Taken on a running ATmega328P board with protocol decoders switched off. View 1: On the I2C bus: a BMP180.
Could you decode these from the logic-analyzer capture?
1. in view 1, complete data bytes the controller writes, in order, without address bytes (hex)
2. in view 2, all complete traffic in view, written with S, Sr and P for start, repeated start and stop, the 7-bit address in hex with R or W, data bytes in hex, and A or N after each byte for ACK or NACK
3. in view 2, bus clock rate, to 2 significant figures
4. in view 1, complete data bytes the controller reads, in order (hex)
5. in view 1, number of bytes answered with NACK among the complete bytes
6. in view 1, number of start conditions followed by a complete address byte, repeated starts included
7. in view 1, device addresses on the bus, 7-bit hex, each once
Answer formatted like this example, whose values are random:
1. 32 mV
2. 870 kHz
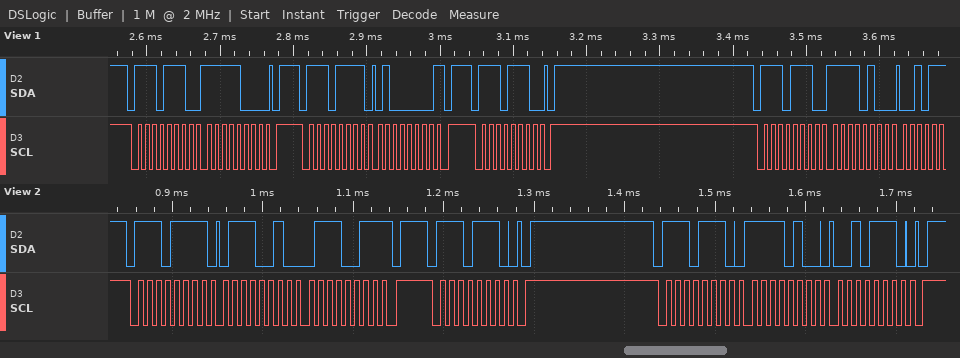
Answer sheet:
1. F8 F4
2. S 77R A 72 A 73 N P S 77W A P S 77W A F4 A 2E A P
3. 100 kHz
4. 40
5. 1
6. 4
7. 0x77
